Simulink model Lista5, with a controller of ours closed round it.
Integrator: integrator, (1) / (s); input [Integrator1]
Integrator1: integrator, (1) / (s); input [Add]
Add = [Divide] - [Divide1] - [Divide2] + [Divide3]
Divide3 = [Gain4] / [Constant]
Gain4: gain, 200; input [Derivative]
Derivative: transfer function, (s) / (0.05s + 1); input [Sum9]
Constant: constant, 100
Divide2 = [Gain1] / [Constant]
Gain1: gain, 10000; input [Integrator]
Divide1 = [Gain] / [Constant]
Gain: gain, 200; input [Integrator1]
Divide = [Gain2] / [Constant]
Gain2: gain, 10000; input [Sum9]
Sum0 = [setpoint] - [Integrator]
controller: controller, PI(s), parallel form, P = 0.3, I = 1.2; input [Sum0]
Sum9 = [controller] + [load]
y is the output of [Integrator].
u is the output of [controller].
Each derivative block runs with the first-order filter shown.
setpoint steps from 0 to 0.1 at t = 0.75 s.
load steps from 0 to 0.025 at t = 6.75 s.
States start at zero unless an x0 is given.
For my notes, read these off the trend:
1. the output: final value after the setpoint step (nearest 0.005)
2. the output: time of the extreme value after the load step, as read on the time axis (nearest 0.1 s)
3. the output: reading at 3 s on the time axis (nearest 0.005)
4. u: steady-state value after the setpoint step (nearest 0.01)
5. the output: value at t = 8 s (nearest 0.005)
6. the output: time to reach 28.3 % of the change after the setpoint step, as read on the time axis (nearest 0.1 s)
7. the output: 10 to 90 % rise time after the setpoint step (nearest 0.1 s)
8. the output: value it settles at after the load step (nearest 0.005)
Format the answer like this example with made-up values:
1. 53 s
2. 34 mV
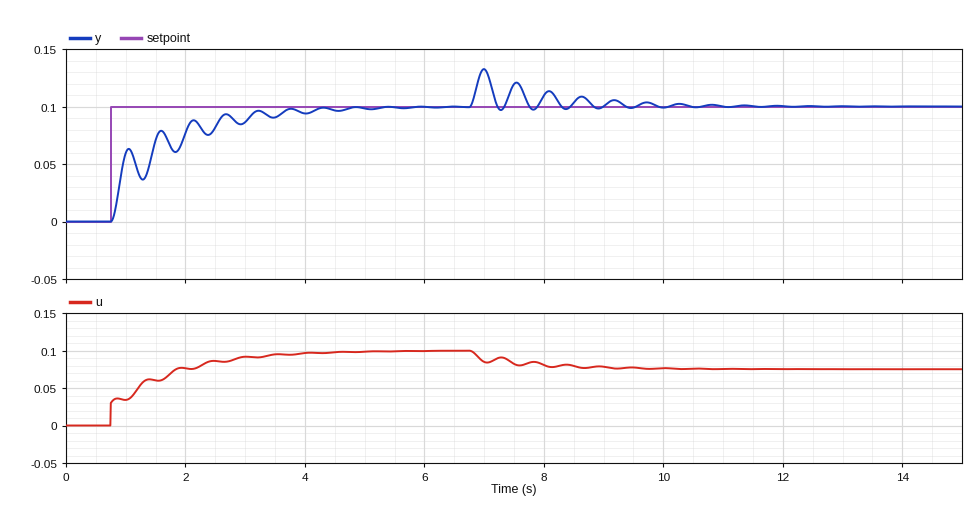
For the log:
1. 0.100
2. 7.0 s
3. 0.085
4. 0.10
5. 0.110
6. 0.9 s
7. 1.8 s
8. 0.100
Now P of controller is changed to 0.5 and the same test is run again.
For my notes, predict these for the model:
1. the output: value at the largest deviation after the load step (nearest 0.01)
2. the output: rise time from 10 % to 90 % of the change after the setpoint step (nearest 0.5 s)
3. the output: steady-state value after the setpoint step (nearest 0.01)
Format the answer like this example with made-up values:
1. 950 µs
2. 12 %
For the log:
1. 0.13
2. 1.5 s
3. 0.10
